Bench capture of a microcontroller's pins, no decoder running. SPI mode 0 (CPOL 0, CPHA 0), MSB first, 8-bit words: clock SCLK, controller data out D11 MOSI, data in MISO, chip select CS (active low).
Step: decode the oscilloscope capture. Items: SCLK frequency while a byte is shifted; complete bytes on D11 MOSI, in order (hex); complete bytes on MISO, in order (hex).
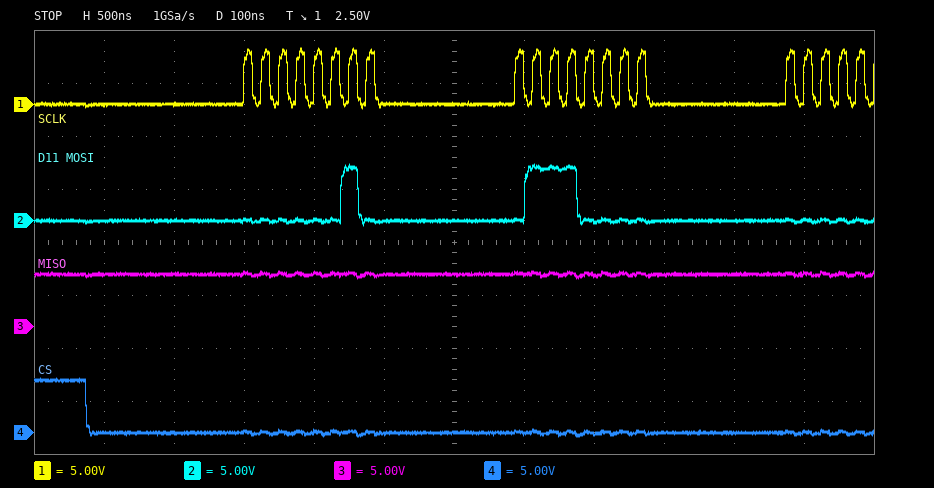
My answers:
8 MHz
0x02 0x70
0xFF 0xFF
